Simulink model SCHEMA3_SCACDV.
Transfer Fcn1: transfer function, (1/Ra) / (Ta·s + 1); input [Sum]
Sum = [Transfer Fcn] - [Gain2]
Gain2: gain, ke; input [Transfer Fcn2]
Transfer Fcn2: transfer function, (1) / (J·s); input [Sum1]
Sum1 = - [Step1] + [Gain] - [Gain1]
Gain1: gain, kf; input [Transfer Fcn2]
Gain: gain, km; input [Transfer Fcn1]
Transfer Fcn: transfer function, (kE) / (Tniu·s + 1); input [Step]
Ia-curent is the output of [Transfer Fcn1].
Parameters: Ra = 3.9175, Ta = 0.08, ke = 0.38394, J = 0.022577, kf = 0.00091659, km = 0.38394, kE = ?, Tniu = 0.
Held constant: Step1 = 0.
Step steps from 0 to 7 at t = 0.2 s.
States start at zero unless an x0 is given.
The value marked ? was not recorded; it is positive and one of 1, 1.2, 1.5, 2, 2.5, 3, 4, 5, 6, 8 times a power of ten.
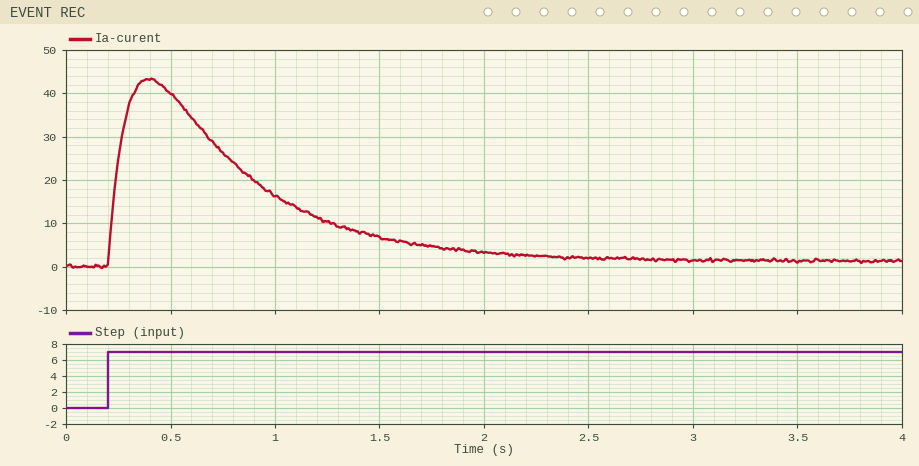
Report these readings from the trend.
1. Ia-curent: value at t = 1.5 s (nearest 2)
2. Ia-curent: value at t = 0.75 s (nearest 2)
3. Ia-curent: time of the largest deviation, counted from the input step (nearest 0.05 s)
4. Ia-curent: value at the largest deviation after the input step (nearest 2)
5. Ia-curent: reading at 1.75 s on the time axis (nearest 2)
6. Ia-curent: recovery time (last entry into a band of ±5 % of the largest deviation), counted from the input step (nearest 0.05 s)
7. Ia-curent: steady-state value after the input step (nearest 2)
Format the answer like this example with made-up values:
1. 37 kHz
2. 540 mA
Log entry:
1. 6
2. 26
3. 0.20 s
4. 44
5. 4
6. 1.75 s
7. 2
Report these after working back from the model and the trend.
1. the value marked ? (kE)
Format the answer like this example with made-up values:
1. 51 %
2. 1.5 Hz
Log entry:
1. 30
